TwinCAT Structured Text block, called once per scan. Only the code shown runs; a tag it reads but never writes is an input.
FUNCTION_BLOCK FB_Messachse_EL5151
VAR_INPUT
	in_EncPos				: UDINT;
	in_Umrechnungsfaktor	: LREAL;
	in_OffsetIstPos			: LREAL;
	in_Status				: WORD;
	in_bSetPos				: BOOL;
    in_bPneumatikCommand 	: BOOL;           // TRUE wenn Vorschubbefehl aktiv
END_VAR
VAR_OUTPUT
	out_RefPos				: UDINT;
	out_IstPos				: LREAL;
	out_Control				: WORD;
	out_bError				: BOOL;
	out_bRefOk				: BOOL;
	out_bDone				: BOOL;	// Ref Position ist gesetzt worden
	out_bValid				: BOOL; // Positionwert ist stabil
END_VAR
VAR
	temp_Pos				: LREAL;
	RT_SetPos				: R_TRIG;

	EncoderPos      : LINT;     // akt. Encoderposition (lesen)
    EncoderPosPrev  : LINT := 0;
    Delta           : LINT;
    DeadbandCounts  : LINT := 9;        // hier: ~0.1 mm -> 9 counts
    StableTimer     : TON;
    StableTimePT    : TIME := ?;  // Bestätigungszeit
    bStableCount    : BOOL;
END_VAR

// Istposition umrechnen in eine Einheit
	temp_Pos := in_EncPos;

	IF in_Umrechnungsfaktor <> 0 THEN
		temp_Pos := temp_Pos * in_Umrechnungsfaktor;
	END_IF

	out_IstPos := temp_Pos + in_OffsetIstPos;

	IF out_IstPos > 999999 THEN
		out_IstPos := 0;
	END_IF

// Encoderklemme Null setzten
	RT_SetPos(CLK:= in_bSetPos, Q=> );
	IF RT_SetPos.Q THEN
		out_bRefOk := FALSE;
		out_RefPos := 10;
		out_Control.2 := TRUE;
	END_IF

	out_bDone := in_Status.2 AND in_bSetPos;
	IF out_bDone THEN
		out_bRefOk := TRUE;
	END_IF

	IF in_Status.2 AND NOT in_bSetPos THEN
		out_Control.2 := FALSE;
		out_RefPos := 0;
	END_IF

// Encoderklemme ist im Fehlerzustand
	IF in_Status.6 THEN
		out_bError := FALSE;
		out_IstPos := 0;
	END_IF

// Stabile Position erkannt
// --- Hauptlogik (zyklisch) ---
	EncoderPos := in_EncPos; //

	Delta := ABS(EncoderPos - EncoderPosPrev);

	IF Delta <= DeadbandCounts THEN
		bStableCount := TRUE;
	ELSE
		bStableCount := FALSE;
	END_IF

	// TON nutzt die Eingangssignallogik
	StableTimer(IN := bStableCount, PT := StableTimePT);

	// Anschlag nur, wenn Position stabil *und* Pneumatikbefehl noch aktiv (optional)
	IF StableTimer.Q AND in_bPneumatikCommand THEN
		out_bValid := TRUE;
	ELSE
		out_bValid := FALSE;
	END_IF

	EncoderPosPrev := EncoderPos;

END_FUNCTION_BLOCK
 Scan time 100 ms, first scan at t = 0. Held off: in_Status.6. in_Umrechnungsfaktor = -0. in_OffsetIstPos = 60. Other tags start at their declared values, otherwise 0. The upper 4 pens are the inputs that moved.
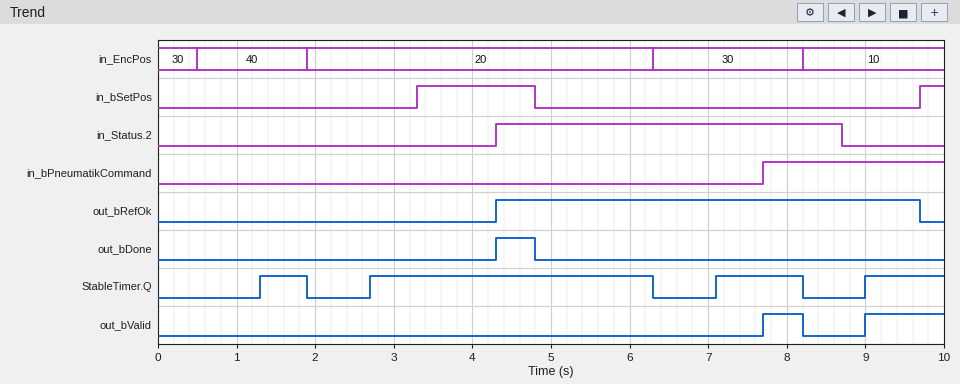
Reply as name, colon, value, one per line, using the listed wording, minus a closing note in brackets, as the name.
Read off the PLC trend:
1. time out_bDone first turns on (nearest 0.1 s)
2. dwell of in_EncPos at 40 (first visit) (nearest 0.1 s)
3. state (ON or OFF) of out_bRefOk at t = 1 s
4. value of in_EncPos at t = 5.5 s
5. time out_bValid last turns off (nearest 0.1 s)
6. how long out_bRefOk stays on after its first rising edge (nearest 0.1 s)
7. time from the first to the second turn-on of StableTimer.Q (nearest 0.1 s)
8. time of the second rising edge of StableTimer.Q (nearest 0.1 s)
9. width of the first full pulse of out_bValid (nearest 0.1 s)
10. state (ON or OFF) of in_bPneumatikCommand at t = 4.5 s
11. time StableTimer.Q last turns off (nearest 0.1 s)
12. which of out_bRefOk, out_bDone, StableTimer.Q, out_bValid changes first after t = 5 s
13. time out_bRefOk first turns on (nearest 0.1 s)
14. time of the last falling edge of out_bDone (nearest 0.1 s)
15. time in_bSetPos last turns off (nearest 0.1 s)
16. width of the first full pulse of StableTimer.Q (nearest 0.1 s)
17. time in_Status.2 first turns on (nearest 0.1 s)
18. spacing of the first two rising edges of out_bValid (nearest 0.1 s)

time out_bDone first turns on: 4.3 s
dwell of in_EncPos at 40 (first visit): 1.4 s
state (ON or OFF) of out_bRefOk at t = 1 s: OFF
value of in_EncPos at t = 5.5 s: 20
time out_bValid last turns off: 8.2 s
how long out_bRefOk stays on after its first rising edge: 5.4 s
time from the first to the second turn-on of StableTimer.Q: 1.4 s
time of the second rising edge of StableTimer.Q: 2.7 s
width of the first full pulse of out_bValid: 0.5 s
state (ON or OFF) of in_bPneumatikCommand at t = 4.5 s: OFF
time StableTimer.Q last turns off: 8.2 s
which of out_bRefOk, out_bDone, StableTimer.Q, out_bValid changes first after t = 5 s: StableTimer.Q
time out_bRefOk first turns on: 4.3 s
time of the last falling edge of out_bDone: 4.8 s
time in_bSetPos last turns off: 4.8 s
width of the first full pulse of StableTimer.Q: 0.6 s
time in_Status.2 first turns on: 4.3 s
spacing of the first two rising edges of out_bValid: 1.3 s
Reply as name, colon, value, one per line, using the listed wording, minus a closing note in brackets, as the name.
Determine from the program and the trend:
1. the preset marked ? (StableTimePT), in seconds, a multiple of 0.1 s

the preset marked ? (StableTimePT), in seconds, a multiple of 0.1 s: 0.7 s
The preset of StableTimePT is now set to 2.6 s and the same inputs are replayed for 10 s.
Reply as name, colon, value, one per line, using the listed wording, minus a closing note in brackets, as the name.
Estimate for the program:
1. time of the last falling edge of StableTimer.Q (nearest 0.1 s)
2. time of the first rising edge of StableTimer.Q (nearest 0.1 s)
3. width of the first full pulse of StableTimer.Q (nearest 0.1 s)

time of the last falling edge of StableTimer.Q: 6.3 s
time of the first rising edge of StableTimer.Q: 4.6 s
width of the first full pulse of StableTimer.Q: 1.7 s
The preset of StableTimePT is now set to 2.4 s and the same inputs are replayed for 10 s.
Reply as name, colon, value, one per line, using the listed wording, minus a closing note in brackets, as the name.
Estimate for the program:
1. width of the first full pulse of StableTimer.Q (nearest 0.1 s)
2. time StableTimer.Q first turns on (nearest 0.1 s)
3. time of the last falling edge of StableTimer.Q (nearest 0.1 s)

width of the first full pulse of StableTimer.Q: 1.9 s
time StableTimer.Q first turns on: 4.4 s
time of the last falling edge of StableTimer.Q: 6.3 s
